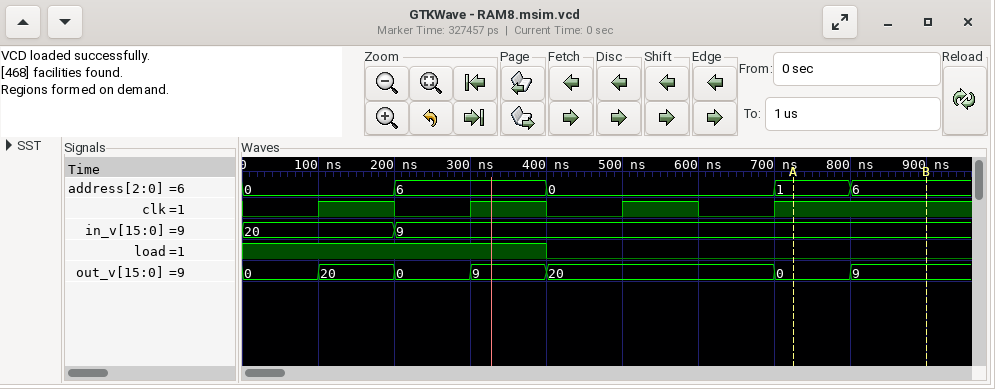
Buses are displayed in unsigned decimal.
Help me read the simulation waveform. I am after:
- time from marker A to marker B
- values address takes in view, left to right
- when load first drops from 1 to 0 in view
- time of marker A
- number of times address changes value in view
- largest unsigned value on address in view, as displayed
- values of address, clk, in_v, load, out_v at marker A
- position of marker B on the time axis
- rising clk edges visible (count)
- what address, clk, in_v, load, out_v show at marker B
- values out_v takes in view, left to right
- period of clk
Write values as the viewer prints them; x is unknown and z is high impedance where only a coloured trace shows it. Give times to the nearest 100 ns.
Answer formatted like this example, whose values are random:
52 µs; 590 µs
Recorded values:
200 ns; 0, 6, 0, 1, 6; 400 ns; 700 ns; 4; 6; address=1, clk=1, in_v=9, load=0, out_v=0; 900 ns; 4; address=6, clk=1, in_v=9, load=0, out_v=9; 0, 20, 0, 9, 20, 0, 9; 200 ns
